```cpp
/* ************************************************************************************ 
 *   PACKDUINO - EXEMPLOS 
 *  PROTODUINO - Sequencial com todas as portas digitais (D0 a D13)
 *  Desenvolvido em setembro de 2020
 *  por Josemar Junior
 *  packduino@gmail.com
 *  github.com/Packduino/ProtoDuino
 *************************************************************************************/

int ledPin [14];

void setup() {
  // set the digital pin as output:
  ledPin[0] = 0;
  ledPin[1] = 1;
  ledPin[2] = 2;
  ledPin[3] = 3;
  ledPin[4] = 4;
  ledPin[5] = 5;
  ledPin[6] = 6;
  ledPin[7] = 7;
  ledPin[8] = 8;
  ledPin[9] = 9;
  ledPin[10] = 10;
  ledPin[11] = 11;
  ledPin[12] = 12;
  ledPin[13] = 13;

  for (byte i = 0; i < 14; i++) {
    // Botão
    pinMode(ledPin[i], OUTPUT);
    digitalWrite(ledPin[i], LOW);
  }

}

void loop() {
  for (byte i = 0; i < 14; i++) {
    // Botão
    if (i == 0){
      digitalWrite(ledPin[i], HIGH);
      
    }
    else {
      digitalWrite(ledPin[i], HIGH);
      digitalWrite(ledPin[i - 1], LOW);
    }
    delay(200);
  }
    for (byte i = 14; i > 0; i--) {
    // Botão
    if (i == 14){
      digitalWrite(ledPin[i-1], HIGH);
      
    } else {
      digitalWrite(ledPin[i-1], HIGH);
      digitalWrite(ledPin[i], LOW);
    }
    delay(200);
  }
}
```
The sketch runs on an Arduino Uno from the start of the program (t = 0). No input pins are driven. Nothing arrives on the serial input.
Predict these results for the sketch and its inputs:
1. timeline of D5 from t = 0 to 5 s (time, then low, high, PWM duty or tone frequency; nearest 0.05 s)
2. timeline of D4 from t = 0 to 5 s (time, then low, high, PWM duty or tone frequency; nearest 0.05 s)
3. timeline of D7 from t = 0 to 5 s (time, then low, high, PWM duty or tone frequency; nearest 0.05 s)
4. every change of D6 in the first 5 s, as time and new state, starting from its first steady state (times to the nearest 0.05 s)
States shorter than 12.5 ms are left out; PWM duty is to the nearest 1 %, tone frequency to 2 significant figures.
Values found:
0 s low; 1 s high; 1.2 s low; 4.4 s high; 4.6 s low
0 s low; 0.8 s high; 1 s low; 4.6 s high; 4.8 s low
0 s low; 1.4 s high; 1.6 s low; 4 s high; 4.2 s low
0 s low; 1.2 s high; 1.4 s low; 4.2 s high; 4.4 s low
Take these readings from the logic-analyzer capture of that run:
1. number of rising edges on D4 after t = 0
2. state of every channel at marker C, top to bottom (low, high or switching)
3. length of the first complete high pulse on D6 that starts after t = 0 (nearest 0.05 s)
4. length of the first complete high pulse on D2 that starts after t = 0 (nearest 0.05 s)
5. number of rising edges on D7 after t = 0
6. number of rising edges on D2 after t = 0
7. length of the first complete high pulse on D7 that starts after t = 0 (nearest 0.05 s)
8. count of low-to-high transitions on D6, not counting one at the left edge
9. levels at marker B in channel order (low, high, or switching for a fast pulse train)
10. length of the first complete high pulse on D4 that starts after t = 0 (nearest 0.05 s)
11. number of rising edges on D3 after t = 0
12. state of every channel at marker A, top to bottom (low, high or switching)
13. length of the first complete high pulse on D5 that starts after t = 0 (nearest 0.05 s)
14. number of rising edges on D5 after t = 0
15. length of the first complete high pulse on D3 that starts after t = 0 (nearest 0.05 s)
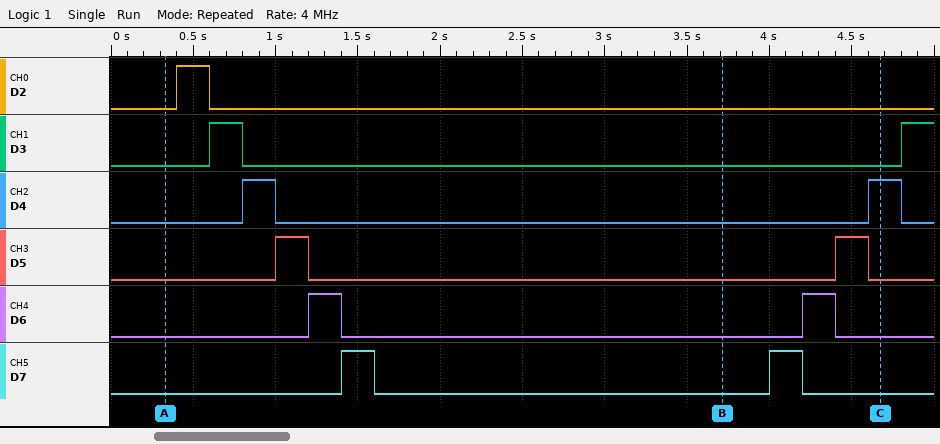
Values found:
2
D2 low, D3 low, D4 high, D5 low, D6 low, D7 low
0.20 s
0.20 s
2
1
0.20 s
2
D2 low, D3 low, D4 low, D5 low, D6 low, D7 low
0.20 s
2
D2 low, D3 low, D4 low, D5 low, D6 low, D7 low
0.20 s
2
0.20 s
